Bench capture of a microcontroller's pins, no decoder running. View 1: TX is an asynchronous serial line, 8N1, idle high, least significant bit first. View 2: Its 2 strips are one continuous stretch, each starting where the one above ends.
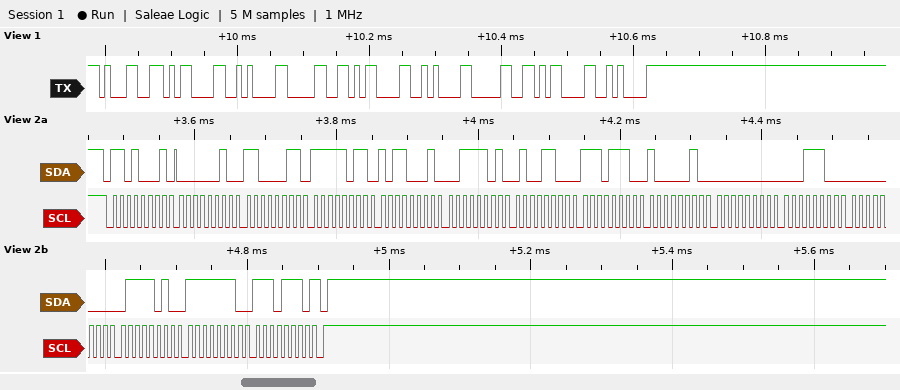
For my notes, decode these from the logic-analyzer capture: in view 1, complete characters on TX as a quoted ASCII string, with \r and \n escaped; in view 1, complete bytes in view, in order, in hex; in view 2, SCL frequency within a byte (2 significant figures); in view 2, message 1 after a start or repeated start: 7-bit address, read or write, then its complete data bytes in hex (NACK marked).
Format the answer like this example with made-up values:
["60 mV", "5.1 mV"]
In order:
["\"1\\r\\n0\\r\\n0\\r\\n\"", "31 0D 0A 30 0D 0A 30 0D 0A", "100 kHz", "0x68 read: 02 C3 FB B1 3D 4C EE 82 00 1C 00 7A FE EE NACK"]
